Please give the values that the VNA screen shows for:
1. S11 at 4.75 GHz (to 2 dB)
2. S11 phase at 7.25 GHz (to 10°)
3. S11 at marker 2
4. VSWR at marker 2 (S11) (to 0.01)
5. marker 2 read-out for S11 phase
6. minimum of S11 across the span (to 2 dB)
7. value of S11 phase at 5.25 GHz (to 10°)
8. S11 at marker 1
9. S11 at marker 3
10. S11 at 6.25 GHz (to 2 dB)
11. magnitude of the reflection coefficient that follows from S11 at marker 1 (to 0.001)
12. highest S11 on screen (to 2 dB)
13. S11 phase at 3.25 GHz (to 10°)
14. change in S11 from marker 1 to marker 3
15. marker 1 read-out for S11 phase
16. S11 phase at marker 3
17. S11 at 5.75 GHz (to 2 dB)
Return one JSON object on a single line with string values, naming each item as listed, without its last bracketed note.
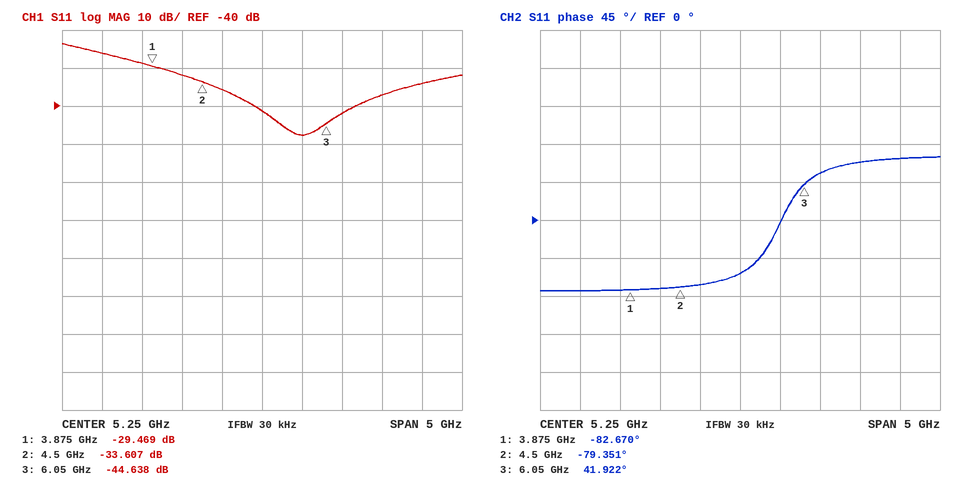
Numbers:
{"S11 at 4.75 GHz": "-36 dB", "S11 phase at 7.25 GHz": "70°", "S11 at marker 2": "-33.607 dB", "VSWR at marker 2 (S11)": "1.04", "marker 2 read-out for S11 phase": "-79.351°", "minimum of S11 across the span": "-48 dB", "value of S11 phase at 5.25 GHz": "-60°", "S11 at marker 1": "-29.469 dB", "S11 at marker 3": "-44.638 dB", "S11 at 6.25 GHz": "-42 dB", "magnitude of the reflection coefficient that follows from S11 at marker 1": "0.034", "highest S11 on screen": "-24 dB", "S11 phase at 3.25 GHz": "-80°", "change in S11 from marker 1 to marker 3": "-15.169 dB", "marker 1 read-out for S11 phase": "-82.670°", "S11 phase at marker 3": "41.922°", "S11 at 5.75 GHz": "-48 dB"}
